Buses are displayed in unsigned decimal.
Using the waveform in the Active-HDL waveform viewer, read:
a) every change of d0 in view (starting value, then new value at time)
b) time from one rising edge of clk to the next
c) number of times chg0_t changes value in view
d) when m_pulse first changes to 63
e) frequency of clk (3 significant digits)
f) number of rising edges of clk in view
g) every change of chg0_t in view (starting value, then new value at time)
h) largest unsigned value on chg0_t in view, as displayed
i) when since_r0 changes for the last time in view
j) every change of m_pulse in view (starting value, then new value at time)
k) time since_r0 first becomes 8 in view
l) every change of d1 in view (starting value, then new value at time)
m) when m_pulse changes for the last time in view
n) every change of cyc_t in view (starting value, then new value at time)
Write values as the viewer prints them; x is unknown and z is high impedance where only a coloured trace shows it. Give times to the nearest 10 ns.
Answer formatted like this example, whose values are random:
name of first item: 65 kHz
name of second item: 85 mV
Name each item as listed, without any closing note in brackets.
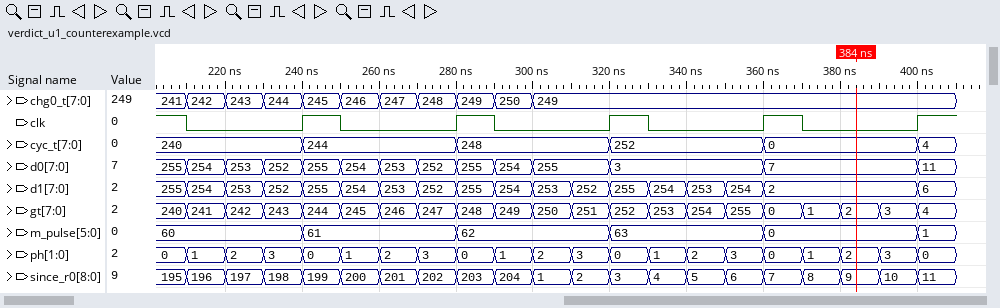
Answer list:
every change of d0 in view: 255, 254 at 210 ns, 253 at 220 ns, 252 at 230 ns, 255 at 240 ns, 254 at 250 ns, 253 at 260 ns, 252 at 270 ns, 255 at 280 ns, 254 at 290 ns, 255 at 300 ns, 3 at 320 ns, 7 at 360 ns, 11 at 400 ns
time from one rising edge of clk to the next: 40 ns
number of times chg0_t changes value in view: 10
when m_pulse first changes to 63: 320 ns
frequency of clk: 25.0 MHz
number of rising edges of clk in view: 5
every change of chg0_t in view: 241, 242 at 210 ns, 243 at 220 ns, 244 at 230 ns, 245 at 240 ns, 246 at 250 ns, 247 at 260 ns, 248 at 270 ns, 249 at 280 ns, 250 at 290 ns, 249 at 300 ns
largest unsigned value on chg0_t in view, as displayed: 250
when since_r0 changes for the last time in view: 400 ns
every change of m_pulse in view: 60, 61 at 240 ns, 62 at 280 ns, 63 at 320 ns, 0 at 360 ns, 1 at 400 ns
time since_r0 first becomes 8 in view: 370 ns
every change of d1 in view: 255, 254 at 210 ns, 253 at 220 ns, 252 at 230 ns, 255 at 240 ns, 254 at 250 ns, 253 at 260 ns, 252 at 270 ns, 255 at 280 ns, 254 at 290 ns, 253 at 300 ns, 252 at 310 ns, 255 at 320 ns, 254 at 330 ns, 253 at 340 ns, 254 at 350 ns, 2 at 360 ns, 6 at 400 ns
when m_pulse changes for the last time in view: 400 ns
every change of cyc_t in view: 240, 244 at 240 ns, 248 at 280 ns, 252 at 320 ns, 0 at 360 ns, 4 at 400 ns
